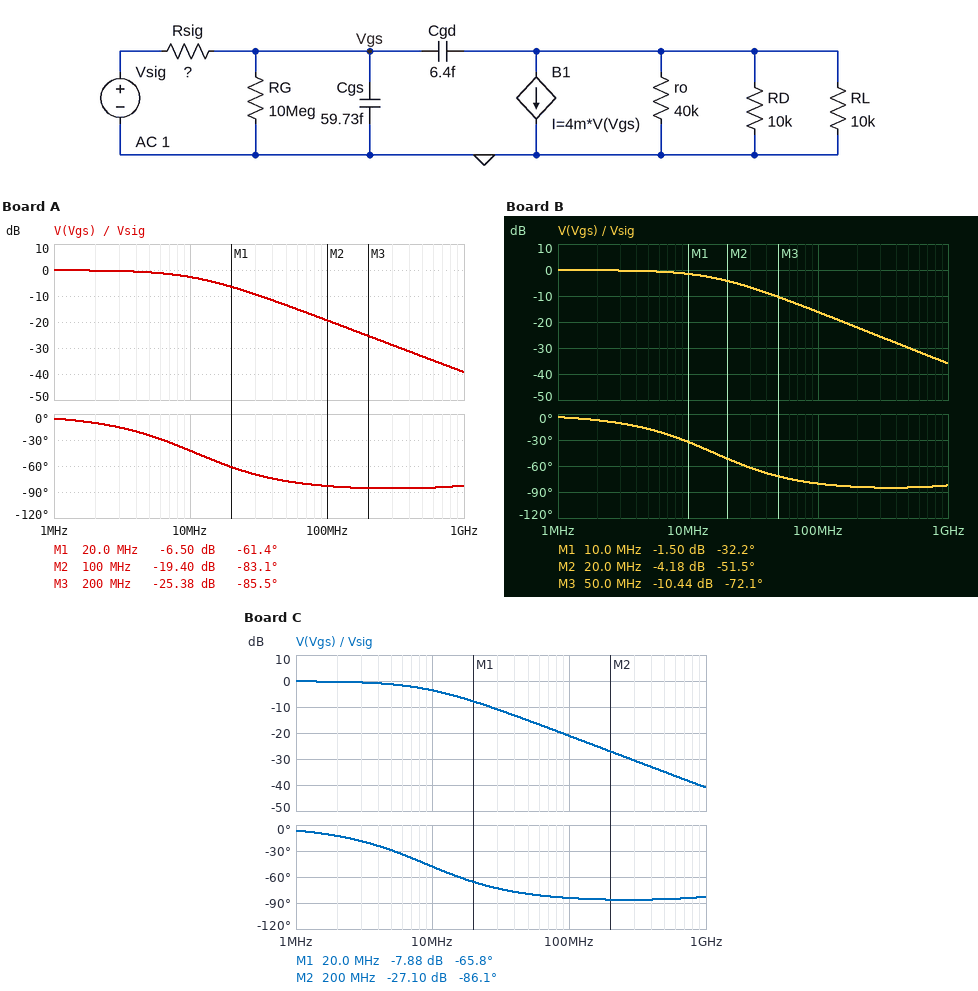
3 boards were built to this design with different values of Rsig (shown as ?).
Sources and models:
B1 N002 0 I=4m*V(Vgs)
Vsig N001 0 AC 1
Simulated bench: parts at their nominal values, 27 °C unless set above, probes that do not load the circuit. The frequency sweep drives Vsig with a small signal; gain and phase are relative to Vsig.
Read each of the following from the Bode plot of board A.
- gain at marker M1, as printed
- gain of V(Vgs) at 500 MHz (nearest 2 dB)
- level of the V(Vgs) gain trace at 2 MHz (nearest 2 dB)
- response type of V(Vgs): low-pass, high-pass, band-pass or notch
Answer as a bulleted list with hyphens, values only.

- -6.50 dB
- -34 dB
- 0 dB
- low-pass
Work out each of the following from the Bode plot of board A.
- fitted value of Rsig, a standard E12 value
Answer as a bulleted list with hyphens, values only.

- 82 kΩ
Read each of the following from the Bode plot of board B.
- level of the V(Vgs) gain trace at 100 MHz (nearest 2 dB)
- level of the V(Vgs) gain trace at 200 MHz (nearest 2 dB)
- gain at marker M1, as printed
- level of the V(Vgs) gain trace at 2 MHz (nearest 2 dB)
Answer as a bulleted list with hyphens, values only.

- -16 dB
- -22 dB
- -1.50 dB
- 0 dB
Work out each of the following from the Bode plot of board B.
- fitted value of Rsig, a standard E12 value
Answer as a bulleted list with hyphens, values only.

- 56 kΩ
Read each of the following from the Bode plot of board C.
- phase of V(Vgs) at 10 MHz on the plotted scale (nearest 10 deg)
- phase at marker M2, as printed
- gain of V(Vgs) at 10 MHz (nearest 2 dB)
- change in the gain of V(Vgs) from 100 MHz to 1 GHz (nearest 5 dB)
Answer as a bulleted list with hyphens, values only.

- -50 deg
- -86.1 deg
- -4 dB
- -20 dB
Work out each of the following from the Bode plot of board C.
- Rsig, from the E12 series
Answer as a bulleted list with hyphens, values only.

- 100 kΩ
